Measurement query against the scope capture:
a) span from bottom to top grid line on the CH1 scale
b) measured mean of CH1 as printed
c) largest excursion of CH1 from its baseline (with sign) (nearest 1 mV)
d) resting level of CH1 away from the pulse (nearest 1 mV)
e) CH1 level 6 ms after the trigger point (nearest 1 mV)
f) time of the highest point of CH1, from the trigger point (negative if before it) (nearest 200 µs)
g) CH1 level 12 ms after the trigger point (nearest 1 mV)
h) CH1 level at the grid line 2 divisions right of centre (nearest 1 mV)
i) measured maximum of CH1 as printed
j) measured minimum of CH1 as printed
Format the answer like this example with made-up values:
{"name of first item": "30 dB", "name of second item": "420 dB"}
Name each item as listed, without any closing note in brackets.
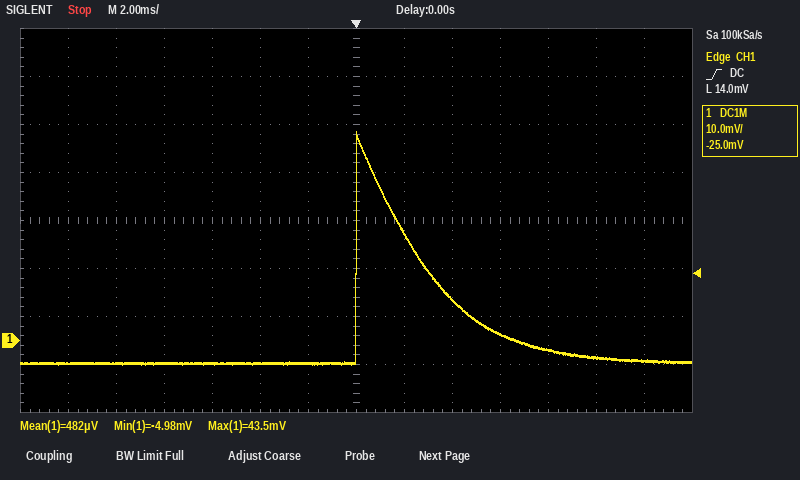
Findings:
{"span from bottom to top grid line on the CH1 scale": "80 mV", "measured mean of CH1 as printed": "482 µV", "largest excursion of CH1 from its baseline (with sign)": "+48 mV", "resting level of CH1 away from the pulse": "-5 mV", "CH1 level 6 ms after the trigger point": "1 mV", "time of the highest point of CH1, from the trigger point (negative if before it)": "0.0 ms", "CH1 level 12 ms after the trigger point": "-4 mV", "CH1 level at the grid line 2 divisions right of centre": "9 mV", "measured maximum of CH1 as printed": "43.5 mV", "measured minimum of CH1 as printed": "-4.98 mV"}
